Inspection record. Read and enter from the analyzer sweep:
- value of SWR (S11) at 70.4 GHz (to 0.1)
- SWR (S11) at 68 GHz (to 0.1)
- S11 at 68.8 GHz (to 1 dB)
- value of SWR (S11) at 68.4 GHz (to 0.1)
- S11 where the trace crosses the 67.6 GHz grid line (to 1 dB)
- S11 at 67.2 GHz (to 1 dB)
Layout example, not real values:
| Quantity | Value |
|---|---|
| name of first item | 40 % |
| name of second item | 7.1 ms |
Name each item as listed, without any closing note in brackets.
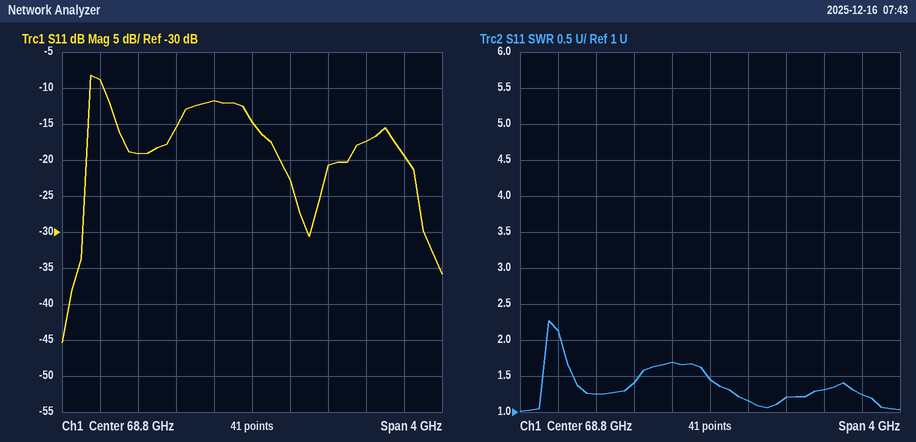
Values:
| Quantity | Value |
|---|---|
| value of SWR (S11) at 70.4 GHz | 1.2 |
| SWR (S11) at 68 GHz | 1.4 |
| S11 at 68.8 GHz | -15 dB |
| value of SWR (S11) at 68.4 GHz | 1.7 |
| S11 where the trace crosses the 67.6 GHz grid line | -19 dB |
| S11 at 67.2 GHz | -9 dB |
